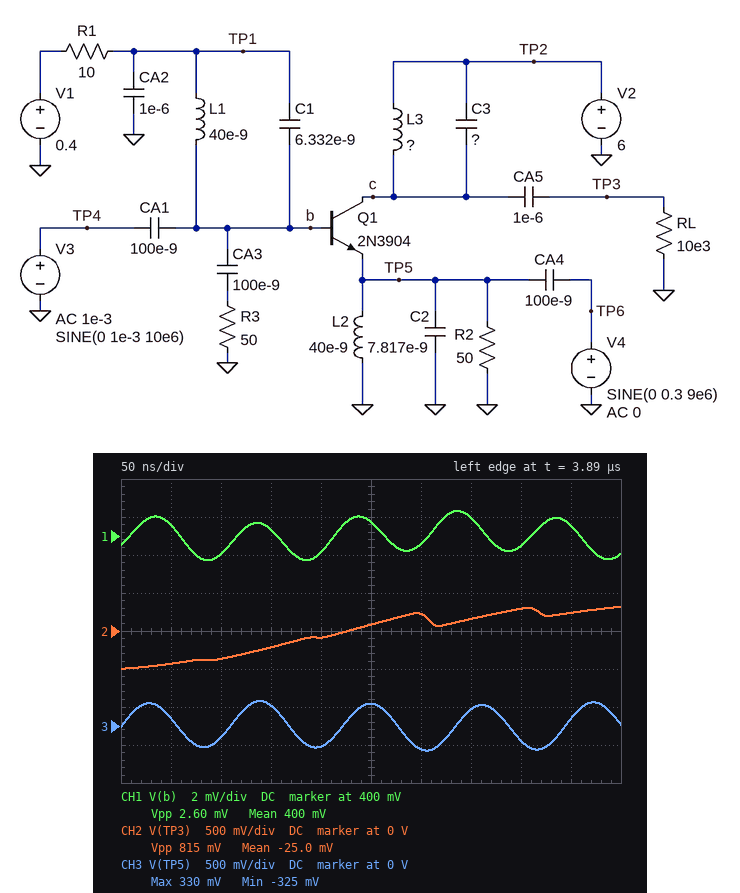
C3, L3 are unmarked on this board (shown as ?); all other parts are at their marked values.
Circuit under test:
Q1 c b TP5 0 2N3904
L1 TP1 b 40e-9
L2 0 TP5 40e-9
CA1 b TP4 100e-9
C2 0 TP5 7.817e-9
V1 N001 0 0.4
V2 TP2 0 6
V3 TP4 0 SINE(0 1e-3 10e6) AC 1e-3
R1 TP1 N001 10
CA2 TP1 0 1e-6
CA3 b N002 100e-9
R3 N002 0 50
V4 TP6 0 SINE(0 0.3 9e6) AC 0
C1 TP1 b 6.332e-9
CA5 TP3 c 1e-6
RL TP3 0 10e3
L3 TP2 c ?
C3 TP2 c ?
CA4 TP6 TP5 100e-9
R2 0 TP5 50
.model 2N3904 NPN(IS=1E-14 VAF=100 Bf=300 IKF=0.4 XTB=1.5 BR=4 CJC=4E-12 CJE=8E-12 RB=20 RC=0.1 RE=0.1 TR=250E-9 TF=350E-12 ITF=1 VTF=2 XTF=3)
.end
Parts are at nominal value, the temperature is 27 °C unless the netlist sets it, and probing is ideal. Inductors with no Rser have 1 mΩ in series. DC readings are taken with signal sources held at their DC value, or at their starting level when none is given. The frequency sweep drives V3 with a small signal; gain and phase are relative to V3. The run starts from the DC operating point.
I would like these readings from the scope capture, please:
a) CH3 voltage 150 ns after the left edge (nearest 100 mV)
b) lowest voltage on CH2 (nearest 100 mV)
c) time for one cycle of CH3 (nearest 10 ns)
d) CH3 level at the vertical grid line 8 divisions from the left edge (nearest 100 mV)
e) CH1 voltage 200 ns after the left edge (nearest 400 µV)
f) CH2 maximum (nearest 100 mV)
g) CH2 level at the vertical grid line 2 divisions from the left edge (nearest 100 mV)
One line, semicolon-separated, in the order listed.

300 mV; -500 mV; 110 ns; -200 mV; 399.2 mV; 300 mV; -400 mV
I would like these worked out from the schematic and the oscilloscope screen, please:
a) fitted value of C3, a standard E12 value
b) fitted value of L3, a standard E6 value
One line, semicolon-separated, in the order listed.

680 pF; 33 µH
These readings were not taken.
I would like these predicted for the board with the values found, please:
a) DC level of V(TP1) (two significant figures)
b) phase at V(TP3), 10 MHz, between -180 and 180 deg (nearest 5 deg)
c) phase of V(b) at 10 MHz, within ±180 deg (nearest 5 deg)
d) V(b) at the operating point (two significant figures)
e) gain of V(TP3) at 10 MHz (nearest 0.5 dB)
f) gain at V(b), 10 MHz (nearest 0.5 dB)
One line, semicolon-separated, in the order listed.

400 mV; 0 deg; 0 deg; 400 mV; -50.5 dB; 0 dB
